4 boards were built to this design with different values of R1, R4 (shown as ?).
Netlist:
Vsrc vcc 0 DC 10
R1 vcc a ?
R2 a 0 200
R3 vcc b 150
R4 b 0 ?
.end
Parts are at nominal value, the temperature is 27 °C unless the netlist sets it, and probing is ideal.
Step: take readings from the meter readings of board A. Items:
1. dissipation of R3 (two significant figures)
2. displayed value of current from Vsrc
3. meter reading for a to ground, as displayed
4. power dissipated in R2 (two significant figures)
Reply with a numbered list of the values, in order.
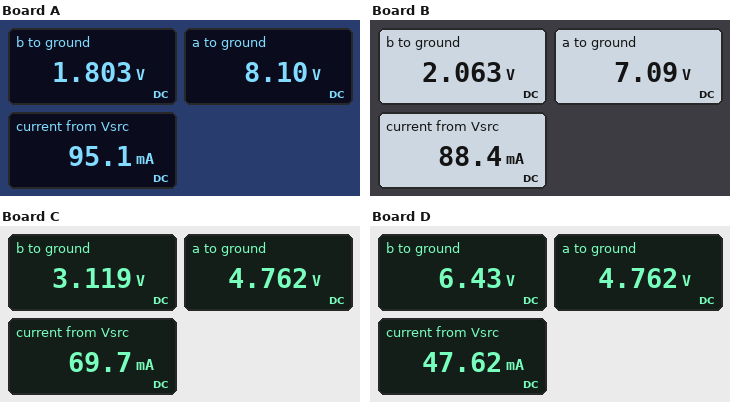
1. 450 mW
2. 95.1 mA
3. 8.10 V
4. 330 mW
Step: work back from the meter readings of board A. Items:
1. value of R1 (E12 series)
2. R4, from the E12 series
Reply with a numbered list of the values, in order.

1. 47 Ω
2. 33 Ω
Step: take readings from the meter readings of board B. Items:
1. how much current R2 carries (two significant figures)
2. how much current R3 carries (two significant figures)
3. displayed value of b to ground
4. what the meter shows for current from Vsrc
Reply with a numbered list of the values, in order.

1. 35 mA
2. 53 mA
3. 2.063 V
4. 88.4 mA
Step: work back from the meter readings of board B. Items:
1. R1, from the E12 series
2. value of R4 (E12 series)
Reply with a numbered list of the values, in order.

1. 82 Ω
2. 39 Ω
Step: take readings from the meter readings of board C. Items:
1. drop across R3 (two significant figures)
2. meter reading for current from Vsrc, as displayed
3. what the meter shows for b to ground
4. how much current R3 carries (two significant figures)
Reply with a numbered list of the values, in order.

1. 6.9 V
2. 69.7 mA
3. 3.119 V
4. 46 mA
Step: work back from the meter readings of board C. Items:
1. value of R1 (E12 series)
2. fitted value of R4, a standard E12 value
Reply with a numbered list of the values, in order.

1. 220 Ω
2. 68 Ω
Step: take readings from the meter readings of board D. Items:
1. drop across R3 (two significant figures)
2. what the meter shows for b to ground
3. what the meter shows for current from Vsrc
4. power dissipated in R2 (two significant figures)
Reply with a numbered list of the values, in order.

1. 3.6 V
2. 6.43 V
3. 47.62 mA
4. 110 mW
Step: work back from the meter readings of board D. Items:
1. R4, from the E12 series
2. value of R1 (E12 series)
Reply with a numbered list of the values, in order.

1. 270 Ω
2. 220 Ω
